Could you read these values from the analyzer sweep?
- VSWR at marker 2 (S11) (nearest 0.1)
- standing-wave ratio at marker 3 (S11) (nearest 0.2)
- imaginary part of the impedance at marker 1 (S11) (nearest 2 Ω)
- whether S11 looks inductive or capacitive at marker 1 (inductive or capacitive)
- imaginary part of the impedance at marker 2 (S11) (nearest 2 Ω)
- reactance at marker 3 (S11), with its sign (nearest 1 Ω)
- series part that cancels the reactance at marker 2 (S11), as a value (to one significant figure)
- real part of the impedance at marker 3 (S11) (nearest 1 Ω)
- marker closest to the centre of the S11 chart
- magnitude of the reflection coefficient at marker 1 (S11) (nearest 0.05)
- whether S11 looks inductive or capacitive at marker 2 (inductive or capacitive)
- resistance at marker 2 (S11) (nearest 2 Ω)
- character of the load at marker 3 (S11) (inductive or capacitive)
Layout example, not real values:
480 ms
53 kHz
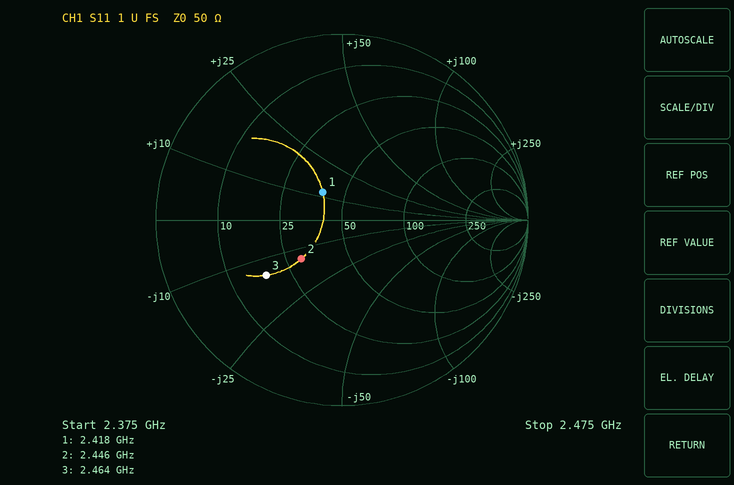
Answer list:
1.9
3.0
+12 Ω
inductive
-14 Ω
-14 Ω
900 pH
18 Ω
marker 1
0.20
capacitive
30 Ω
capacitive
